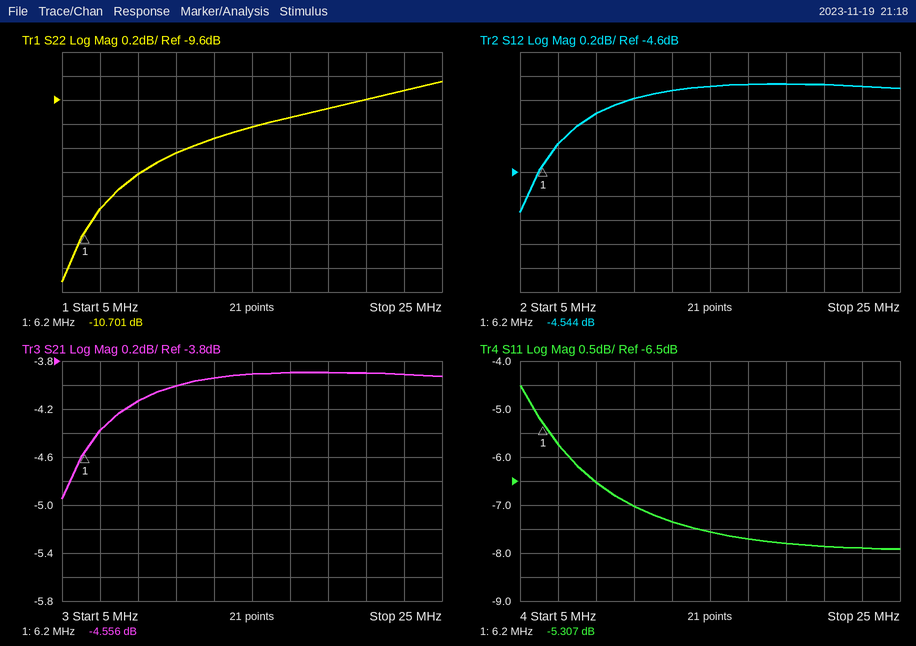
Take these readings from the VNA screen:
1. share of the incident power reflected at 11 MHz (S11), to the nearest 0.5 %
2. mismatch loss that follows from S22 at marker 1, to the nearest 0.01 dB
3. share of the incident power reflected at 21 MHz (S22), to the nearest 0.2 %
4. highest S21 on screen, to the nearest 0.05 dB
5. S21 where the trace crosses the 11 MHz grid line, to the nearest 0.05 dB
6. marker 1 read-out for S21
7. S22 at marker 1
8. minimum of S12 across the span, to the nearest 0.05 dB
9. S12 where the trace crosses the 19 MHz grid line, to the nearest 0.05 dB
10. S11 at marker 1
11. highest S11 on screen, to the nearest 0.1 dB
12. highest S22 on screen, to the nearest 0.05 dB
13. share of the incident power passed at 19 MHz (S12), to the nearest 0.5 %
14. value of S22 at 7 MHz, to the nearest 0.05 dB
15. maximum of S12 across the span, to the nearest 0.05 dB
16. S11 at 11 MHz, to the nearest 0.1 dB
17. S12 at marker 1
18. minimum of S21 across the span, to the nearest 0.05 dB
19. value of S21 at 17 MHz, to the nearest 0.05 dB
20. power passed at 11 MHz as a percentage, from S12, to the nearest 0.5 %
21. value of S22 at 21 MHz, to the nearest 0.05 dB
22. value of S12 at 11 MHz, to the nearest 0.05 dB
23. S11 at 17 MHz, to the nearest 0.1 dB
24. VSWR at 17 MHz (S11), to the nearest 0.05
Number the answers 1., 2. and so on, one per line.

1. 20.0 %
2. 0.39 dB
3. 11.0 %
4. -3.90 dB
5. -4.00 dB
6. -4.556 dB
7. -10.701 dB
8. -4.95 dB
9. -3.85 dB
10. -5.307 dB
11. -4.5 dB
12. -9.45 dB
13. 41.0 %
14. -10.50 dB
15. -3.85 dB
16. -7.0 dB
17. -4.544 dB
18. -4.95 dB
19. -3.90 dB
20. 40.0 %
21. -9.60 dB
22. -4.00 dB
23. -7.7 dB
24. 2.40
